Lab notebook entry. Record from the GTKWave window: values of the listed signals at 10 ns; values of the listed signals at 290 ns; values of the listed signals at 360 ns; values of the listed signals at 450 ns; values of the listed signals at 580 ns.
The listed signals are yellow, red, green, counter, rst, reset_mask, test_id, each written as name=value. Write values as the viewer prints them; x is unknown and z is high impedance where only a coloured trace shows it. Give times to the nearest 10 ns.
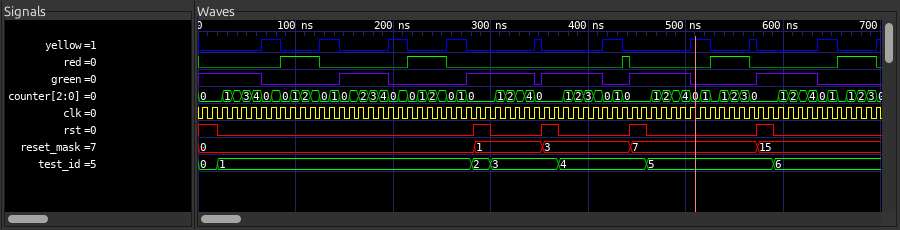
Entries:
yellow=0, red=0, green=1, counter=0, rst=1, reset_mask=0, test_id=0
yellow=0, red=0, green=1, counter=0, rst=1, reset_mask=1, test_id=2
yellow=0, red=0, green=1, counter=0, rst=1, reset_mask=3, test_id=3
yellow=0, red=0, green=1, counter=0, rst=1, reset_mask=7, test_id=4
yellow=0, red=0, green=1, counter=0, rst=1, reset_mask=15, test_id=5
